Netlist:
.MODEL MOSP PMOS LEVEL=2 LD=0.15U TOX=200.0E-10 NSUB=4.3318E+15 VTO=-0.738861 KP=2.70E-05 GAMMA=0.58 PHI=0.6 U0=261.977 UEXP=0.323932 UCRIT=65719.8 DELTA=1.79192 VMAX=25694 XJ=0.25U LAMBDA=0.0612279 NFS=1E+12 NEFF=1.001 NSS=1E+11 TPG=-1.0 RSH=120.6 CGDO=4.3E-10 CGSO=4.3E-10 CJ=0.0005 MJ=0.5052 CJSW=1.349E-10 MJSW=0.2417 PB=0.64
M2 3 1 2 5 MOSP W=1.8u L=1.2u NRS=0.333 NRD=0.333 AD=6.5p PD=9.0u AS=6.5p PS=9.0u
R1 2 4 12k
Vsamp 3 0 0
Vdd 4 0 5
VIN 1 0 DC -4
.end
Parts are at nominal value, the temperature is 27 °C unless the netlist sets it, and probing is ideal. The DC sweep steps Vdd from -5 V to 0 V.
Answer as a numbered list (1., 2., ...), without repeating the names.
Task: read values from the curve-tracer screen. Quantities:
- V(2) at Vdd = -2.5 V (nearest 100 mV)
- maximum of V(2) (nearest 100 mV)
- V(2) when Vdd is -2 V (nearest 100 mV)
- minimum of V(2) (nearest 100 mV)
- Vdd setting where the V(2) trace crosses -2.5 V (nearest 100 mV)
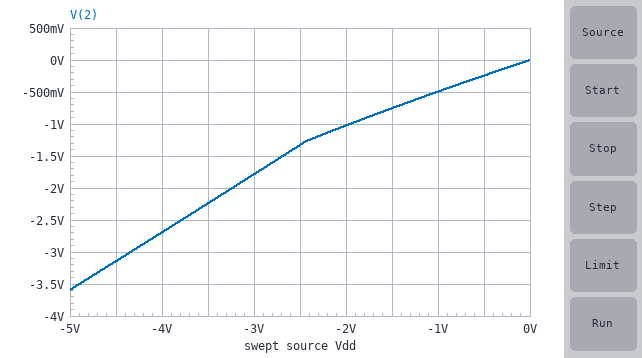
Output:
1. -1.3 V
2. 0 V
3. -1.0 V
4. -3.6 V
5. -3.8 V
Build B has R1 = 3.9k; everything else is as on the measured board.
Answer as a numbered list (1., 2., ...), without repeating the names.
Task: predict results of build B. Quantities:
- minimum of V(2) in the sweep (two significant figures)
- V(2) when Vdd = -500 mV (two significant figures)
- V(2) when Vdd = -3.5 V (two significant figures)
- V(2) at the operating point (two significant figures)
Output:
1. -4.5 V
2. -370 mV
3. -3.1 V
4. 3.8 V
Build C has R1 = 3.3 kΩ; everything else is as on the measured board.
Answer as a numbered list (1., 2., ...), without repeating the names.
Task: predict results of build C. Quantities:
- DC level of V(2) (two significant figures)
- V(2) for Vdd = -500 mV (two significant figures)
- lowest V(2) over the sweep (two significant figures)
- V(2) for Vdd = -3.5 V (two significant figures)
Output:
1. 3.9 V
2. -390 mV
3. -4.6 V
4. -3.1 V
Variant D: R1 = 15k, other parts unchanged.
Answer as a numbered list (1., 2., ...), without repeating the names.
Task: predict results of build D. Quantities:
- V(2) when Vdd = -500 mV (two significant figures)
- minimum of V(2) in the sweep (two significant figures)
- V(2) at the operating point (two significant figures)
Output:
1. -210 mV
2. -3.3 V
3. 2.1 V
